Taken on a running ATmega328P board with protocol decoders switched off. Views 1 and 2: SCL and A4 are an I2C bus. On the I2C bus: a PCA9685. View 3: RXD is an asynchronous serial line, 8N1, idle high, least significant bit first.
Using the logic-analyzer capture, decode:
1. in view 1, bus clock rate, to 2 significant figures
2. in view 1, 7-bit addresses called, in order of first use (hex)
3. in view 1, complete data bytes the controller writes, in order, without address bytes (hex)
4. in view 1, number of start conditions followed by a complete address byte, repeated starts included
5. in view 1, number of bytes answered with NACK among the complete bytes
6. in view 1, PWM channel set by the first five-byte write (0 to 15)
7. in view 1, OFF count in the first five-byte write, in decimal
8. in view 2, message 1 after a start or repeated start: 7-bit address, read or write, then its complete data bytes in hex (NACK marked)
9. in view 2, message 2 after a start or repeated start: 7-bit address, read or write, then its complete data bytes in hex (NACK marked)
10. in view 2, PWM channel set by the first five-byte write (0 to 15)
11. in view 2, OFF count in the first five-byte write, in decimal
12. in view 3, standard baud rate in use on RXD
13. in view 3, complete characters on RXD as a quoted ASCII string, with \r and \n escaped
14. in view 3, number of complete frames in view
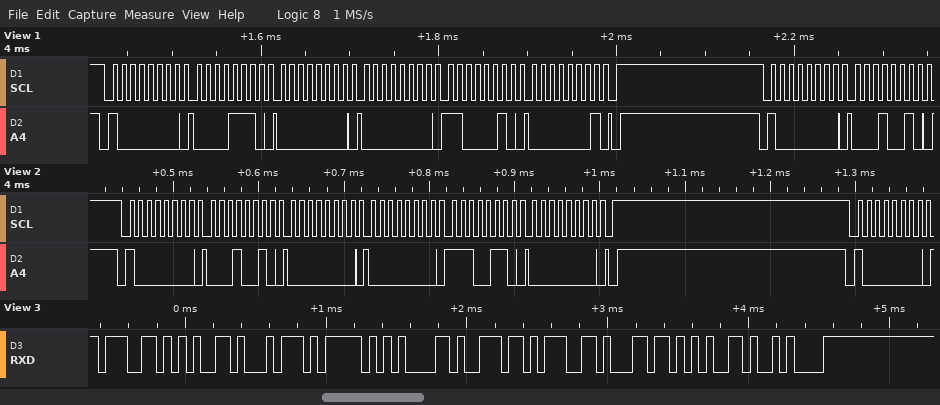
100 kHz
0x40
0E 00 00 C2 01 12
2
0
2
450
0x40 write: 12 00 00 E6 00
0x40 write
3
230
19200 baud
"get_angle\n"
10
